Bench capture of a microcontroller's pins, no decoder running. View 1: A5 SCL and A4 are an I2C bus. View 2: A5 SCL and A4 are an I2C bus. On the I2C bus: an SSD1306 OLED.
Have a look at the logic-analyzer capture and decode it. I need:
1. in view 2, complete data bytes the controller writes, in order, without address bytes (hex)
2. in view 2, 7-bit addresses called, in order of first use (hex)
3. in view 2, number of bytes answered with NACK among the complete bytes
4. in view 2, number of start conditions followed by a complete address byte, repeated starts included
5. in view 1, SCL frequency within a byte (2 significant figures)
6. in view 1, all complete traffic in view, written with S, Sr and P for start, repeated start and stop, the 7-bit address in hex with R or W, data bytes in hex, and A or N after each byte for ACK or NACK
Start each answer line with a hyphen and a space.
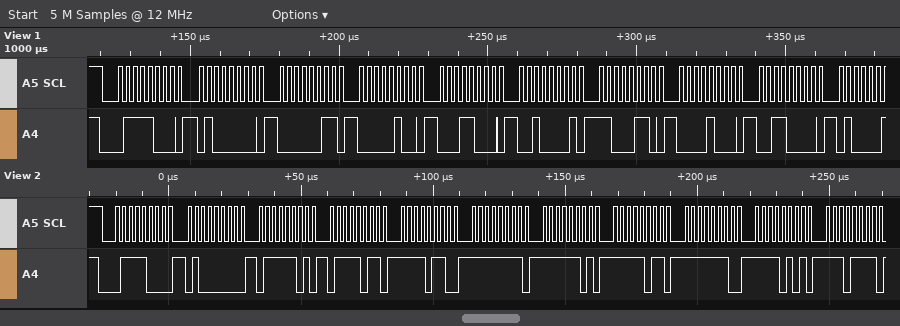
- 40 7D 7B F6 FF FD FB FE F5 EF
- 0x3C
- 0
- 1
- 400 kHz
- S 3CW A 40 A 03 A 04 A 18 A 21 A C6 A 08 A 30 A
